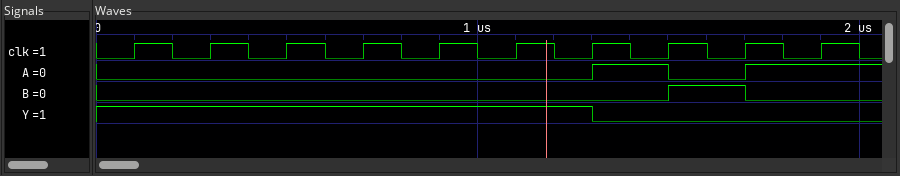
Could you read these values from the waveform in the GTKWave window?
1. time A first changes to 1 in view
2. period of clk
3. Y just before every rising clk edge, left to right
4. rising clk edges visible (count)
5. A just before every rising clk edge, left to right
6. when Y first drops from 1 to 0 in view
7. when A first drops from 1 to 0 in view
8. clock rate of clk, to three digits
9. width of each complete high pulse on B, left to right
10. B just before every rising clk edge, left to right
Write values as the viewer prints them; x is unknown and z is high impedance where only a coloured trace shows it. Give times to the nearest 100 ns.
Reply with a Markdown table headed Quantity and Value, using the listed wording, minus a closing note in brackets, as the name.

| Quantity | Value |
|---|---|
| time A first changes to 1 in view | 1300 ns |
| period of clk | 200 ns |
| Y just before every rising clk edge, left to right | 1 1 1 1 1 1 1 0 0 0 |
| rising clk edges visible | 10 |
| A just before every rising clk edge, left to right | 0 0 0 0 0 0 0 1 0 1 |
| when Y first drops from 1 to 0 in view | 1300 ns |
| when A first drops from 1 to 0 in view | 1500 ns |
| clock rate of clk, to three digits | 5.00 MHz |
| width of each complete high pulse on B, left to right | 200 ns |
| B just before every rising clk edge, left to right | 0 0 0 0 0 0 0 0 1 0 |
